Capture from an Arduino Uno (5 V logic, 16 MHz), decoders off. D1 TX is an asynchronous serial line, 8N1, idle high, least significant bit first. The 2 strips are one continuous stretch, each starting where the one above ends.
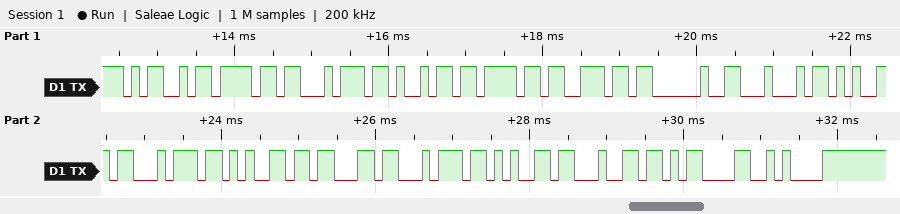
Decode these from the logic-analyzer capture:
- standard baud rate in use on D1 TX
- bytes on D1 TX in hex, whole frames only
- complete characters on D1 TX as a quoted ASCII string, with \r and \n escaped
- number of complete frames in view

9600 baud
0x4D 0x6F 0x74 0x69 0x6F 0x6E 0x20 0x44 0x65 0x74 0x65 0x63 0x74 0x65 0x64 0x0D 0x0A
"Motion Detected\r\n"
17
